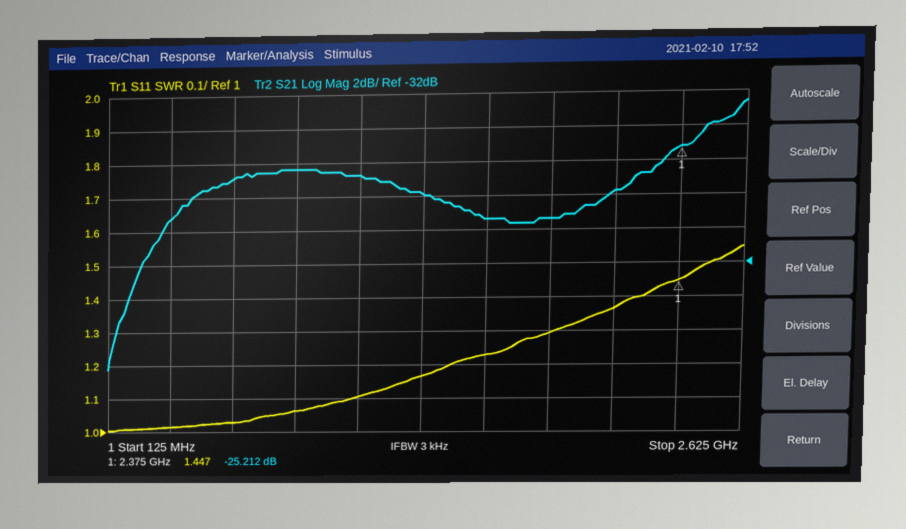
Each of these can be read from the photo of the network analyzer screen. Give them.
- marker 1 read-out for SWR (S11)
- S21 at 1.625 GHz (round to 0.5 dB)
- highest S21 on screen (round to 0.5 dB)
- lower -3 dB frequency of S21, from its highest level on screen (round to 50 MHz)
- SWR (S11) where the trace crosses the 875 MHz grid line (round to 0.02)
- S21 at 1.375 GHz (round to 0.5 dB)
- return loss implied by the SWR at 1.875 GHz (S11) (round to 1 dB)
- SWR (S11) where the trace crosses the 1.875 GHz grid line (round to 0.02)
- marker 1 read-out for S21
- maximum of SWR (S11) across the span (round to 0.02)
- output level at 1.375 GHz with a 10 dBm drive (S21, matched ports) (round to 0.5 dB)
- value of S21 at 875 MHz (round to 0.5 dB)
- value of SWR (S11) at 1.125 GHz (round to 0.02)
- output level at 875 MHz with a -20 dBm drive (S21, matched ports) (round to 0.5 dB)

1.447
-29.5 dB
-22.5 dB
2.35 GHz
1.06
-28.0 dB
18 dB
1.30
-25.212 dB
1.54
-18.0 dBm
-26.5 dB
1.10
-46.5 dBm
